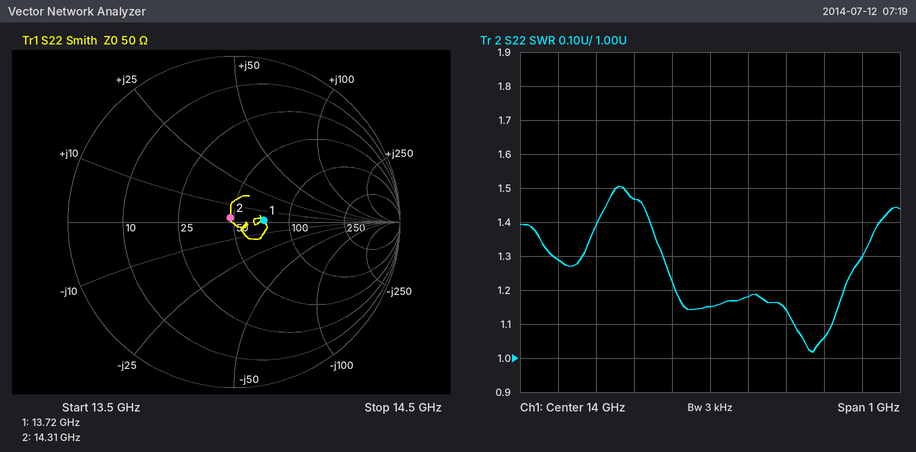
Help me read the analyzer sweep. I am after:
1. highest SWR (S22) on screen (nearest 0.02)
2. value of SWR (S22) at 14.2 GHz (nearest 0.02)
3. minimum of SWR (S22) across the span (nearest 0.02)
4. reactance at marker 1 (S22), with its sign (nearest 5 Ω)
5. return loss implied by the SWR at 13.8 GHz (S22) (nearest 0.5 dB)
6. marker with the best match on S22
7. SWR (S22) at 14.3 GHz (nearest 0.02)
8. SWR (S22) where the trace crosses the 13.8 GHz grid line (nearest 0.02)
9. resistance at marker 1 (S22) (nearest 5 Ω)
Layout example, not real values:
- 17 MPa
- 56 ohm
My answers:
- 1.50
- 1.14
- 1.02
- 0 Ω
- 14.5 dB
- marker 2
- 1.06
- 1.46
- 70 Ω
